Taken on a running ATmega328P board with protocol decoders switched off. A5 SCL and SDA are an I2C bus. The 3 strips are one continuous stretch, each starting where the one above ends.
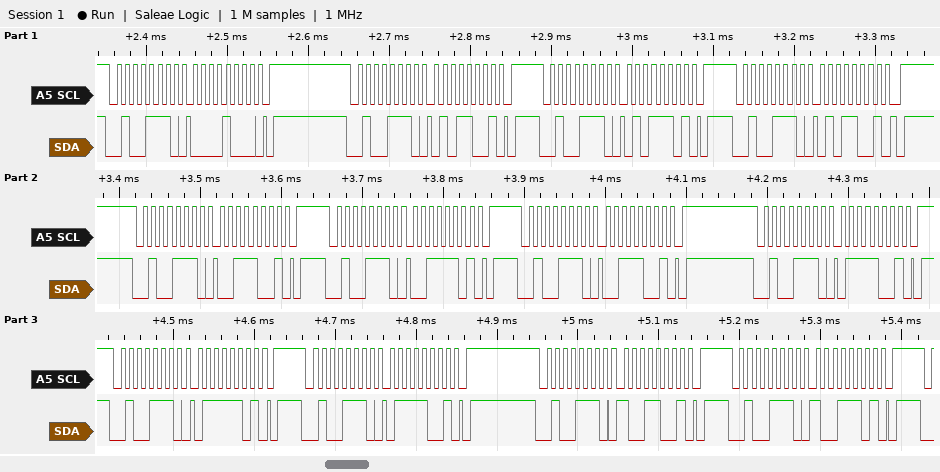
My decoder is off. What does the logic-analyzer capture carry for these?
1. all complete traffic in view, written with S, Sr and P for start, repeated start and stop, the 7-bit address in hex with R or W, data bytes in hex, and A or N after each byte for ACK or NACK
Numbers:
S 27W A 08 A P S 27W A 59 A P S 27W A 5D A P S 27W A 59 A P S 27W A 39 A P S 27W A 3D A P S 27W A 39 A P S 27W A 79 A P S 27W A 7D A P S 27W A 79 A P S 27W A 99 A P S 27W A 9D A P
